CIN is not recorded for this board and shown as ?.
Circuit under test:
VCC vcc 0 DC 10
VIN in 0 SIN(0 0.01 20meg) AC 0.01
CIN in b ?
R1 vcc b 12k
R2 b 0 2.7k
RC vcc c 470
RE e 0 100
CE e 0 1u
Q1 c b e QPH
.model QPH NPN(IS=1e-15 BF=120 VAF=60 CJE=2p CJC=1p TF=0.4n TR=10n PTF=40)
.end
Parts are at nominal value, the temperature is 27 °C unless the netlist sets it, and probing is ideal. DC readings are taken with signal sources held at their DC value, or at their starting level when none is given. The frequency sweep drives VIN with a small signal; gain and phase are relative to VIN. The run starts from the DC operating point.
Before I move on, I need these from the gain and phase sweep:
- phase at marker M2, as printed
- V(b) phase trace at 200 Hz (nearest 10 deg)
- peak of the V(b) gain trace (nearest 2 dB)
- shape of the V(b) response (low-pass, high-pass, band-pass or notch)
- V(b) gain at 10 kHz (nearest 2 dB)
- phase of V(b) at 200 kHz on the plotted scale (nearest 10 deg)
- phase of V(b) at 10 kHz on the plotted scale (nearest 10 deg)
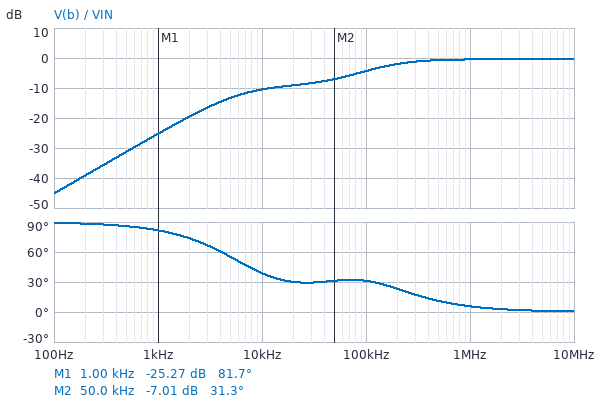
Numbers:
31.3 deg
90 deg
0 dB
high-pass
-10 dB
20 deg
40 deg
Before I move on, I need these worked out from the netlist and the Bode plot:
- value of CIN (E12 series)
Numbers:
4.7 nF
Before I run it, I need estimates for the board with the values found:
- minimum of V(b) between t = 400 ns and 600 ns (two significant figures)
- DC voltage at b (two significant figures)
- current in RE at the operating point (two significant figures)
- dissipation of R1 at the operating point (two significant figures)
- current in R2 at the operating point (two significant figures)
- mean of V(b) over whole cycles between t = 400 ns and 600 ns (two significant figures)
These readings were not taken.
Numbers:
1.7 V
1.7 V
9.1 mA
5.8 mW
620 µA
1.7 V
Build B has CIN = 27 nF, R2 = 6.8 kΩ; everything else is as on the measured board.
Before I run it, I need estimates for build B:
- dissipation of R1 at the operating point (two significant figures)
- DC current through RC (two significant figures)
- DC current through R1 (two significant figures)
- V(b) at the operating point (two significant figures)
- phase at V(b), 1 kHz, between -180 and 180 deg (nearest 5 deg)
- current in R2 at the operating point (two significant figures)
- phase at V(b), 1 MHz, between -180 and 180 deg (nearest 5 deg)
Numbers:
4.6 mW
17 mA
620 µA
2.5 V
65 deg
370 µA
55 deg
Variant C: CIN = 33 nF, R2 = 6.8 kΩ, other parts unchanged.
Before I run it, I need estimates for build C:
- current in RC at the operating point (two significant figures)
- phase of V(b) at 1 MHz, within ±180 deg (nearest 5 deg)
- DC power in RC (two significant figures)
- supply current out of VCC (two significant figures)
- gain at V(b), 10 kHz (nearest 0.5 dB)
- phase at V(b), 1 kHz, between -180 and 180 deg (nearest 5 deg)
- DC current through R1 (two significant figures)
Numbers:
17 mA
50 deg
140 mW
18 mA
-26.0 dB
65 deg
620 µA
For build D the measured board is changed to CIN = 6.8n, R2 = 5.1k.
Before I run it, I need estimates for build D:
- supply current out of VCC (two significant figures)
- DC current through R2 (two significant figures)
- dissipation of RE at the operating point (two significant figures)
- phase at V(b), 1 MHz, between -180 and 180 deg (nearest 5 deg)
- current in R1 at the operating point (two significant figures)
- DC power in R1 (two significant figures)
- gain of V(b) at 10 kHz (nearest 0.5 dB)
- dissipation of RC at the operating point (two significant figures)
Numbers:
17 mA
490 µA
29 mW
5 deg
630 µA
4.7 mW
-8.0 dB
130 mW
